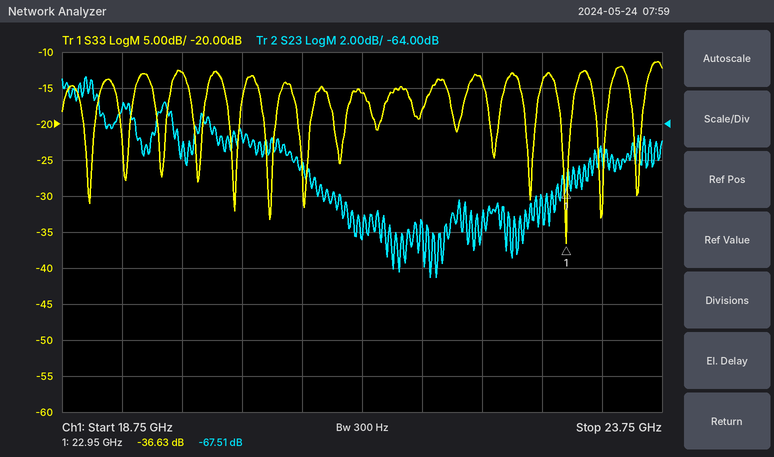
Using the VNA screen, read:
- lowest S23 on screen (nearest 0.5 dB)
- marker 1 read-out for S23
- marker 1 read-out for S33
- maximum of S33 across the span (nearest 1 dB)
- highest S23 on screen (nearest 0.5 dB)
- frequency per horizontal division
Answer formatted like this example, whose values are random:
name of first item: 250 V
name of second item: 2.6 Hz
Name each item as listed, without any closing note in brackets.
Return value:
lowest S23 on screen: -72.5 dB
marker 1 read-out for S23: -67.51 dB
marker 1 read-out for S33: -36.63 dB
maximum of S33 across the span: -11 dB
highest S23 on screen: -61.5 dB
frequency per horizontal division: 500 MHz
